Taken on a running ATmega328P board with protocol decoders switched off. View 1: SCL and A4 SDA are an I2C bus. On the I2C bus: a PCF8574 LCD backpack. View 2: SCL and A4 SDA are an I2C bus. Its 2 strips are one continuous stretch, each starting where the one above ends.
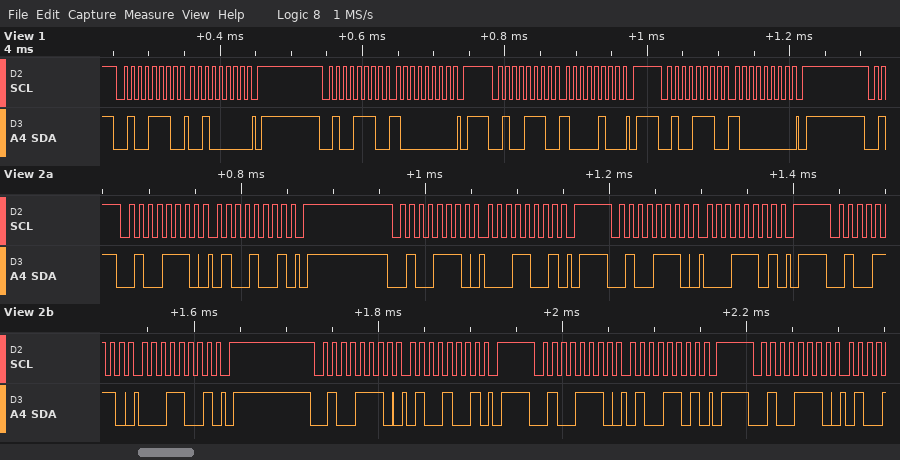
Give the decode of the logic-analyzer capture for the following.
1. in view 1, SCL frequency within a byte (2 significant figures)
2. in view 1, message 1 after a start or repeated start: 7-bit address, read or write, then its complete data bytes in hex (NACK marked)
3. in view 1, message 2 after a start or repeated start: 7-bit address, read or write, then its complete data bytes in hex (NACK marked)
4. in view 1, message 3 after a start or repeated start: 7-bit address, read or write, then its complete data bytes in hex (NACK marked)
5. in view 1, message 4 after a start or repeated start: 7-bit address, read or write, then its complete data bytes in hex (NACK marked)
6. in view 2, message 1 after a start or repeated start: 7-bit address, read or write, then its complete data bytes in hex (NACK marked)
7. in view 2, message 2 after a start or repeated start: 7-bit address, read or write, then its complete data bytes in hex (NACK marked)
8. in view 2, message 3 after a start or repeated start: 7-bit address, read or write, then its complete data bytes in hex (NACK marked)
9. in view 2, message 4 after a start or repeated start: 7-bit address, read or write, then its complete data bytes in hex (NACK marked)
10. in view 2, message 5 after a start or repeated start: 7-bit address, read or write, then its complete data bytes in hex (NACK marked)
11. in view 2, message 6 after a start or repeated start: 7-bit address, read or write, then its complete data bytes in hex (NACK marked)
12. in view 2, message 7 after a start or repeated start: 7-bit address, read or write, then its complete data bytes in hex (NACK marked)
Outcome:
100 kHz
0x27 write: 20
0x27 write: 80
0x27 write: 84
0x27 write: 80
0x27 write: 49
0x27 write: 19
0x27 write: 1D
0x27 write: 19
0x27 write: 49
0x27 write: 4D
0x27 write
